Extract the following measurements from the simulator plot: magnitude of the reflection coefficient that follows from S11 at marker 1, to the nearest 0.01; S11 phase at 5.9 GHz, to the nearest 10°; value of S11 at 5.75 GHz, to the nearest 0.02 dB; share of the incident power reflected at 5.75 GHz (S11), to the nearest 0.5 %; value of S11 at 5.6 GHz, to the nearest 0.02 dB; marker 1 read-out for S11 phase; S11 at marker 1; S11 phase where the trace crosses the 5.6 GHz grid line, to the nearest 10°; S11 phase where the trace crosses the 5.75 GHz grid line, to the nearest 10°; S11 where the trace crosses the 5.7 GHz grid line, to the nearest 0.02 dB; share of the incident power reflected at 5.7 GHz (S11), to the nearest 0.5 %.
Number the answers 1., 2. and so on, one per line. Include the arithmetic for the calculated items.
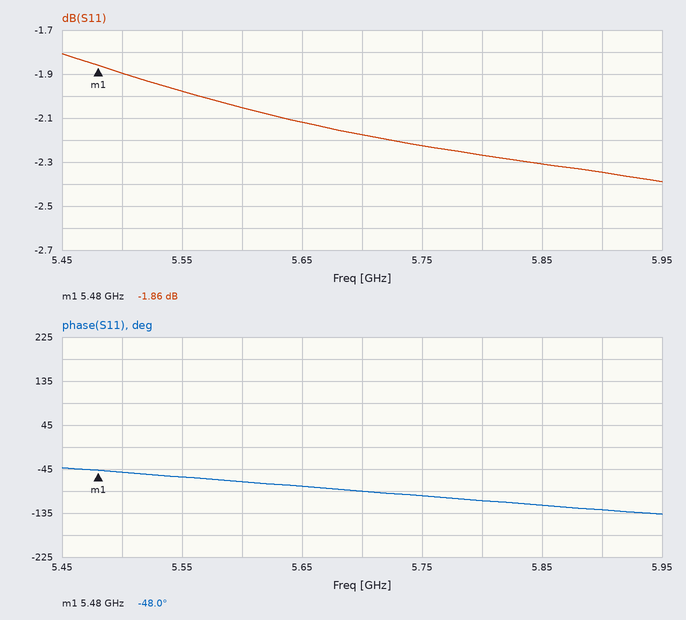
1. 10^(-1.86/20) ≈ 0.81
2. -130°
3. -2.22 dB
4. 10^(-2.22/10) ≈ 60.0 %
5. -2.06 dB
6. -48.0°
7. -1.86 dB
8. -70°
9. -100°
10. -2.18 dB
11. 10^(-2.18/10) ≈ 60.5 %
